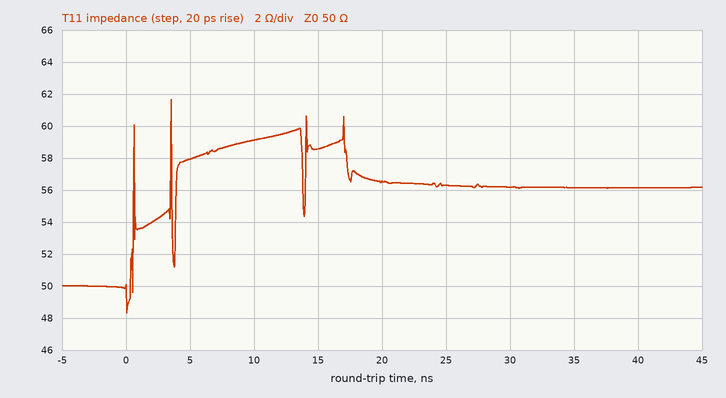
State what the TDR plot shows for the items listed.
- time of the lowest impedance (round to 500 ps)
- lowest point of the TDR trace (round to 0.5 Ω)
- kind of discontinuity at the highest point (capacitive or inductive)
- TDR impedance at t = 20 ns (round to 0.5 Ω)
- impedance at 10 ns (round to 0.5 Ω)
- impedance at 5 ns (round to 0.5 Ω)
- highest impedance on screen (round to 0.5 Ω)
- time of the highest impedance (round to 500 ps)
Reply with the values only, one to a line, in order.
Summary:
0.0 ns
48.5 Ω
inductive
56.5 Ω
59.0 Ω
58.0 Ω
61.5 Ω
3.5 ns
